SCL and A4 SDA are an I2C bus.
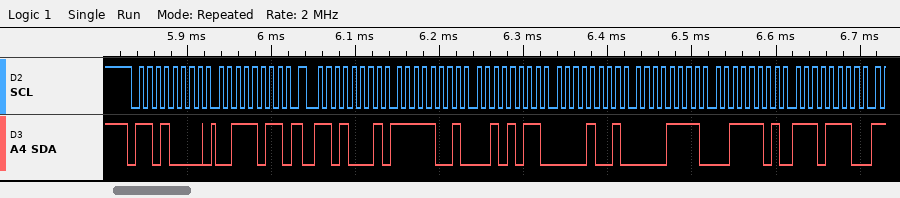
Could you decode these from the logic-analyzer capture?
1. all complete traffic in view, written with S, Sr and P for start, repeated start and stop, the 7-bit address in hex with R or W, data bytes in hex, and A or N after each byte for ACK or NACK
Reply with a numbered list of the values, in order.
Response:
1. S 68W A 3B A Sr 68R A F9 A 2B A 09 A 0F A 3D A EE A
